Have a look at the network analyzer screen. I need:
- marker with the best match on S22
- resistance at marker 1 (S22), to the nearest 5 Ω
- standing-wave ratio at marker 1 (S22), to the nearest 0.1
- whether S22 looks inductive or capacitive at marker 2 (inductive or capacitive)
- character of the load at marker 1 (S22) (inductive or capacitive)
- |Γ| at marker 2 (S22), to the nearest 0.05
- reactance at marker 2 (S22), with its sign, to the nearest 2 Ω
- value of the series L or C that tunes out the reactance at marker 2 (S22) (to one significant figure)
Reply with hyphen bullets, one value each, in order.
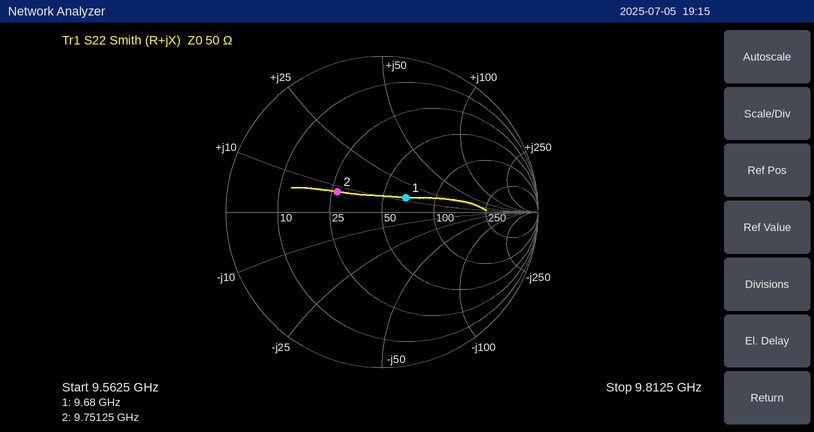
- marker 1
- 65 Ω
- 1.4
- inductive
- inductive
- 0.30
- +8 Ω
- 2 pF
